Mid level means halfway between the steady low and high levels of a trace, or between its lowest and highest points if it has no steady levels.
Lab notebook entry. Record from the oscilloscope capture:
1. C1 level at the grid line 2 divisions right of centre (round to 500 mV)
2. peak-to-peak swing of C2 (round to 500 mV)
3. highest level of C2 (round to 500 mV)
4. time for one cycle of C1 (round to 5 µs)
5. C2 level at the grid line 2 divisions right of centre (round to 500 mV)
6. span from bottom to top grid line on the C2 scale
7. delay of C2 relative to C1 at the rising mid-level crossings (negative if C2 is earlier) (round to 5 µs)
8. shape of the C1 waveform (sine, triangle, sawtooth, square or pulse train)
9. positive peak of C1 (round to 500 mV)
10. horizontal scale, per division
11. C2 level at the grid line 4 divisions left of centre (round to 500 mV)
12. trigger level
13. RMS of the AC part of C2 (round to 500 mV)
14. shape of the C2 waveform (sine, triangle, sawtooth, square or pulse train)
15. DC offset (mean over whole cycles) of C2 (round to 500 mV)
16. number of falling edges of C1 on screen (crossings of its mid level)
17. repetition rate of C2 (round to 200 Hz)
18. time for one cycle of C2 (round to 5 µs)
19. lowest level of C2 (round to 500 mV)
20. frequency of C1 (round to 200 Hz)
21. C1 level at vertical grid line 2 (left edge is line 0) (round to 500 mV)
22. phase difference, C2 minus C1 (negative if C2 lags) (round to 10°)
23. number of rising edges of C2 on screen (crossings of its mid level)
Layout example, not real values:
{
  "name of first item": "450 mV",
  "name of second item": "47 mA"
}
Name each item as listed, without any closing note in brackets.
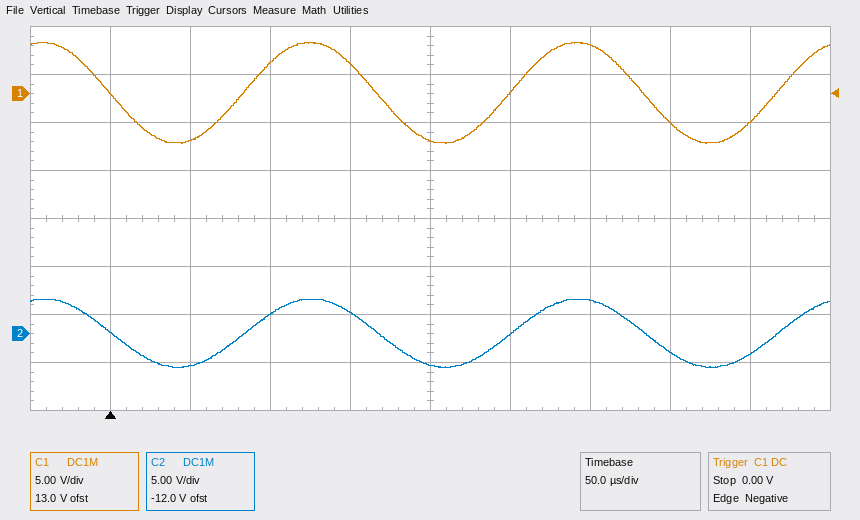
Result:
{
  "C1 level at the grid line 2 divisions right of centre": "5.0 V",
  "peak-to-peak swing of C2": "7.0 V",
  "highest level of C2": "3.5 V",
  "time for one cycle of C1": "165 µs",
  "C2 level at the grid line 2 divisions right of centre": "3.5 V",
  "span from bottom to top grid line on the C2 scale": "40 V",
  "delay of C2 relative to C1 at the rising mid-level crossings (negative if C2 is earlier)": "0 µs",
  "shape of the C1 waveform": "sine",
  "positive peak of C1": "5.5 V",
  "horizontal scale, per division": "50 µs",
  "C2 level at the grid line 4 divisions left of centre": "0.0 V",
  "trigger level": "0.00 V",
  "RMS of the AC part of C2": "2.5 V",
  "shape of the C2 waveform": "sine",
  "DC offset (mean over whole cycles) of C2": "0.0 V",
  "number of falling edges of C1 on screen": "3",
  "repetition rate of C2": "6.0 kHz",
  "time for one cycle of C2": "165 µs",
  "lowest level of C2": "-3.5 V",
  "frequency of C1": "6.0 kHz",
  "C1 level at vertical grid line 2 (left edge is line 0)": "-5.0 V",
  "phase difference, C2 minus C1 (negative if C2 lags)": "0°",
  "number of rising edges of C2 on screen": "3"
}
